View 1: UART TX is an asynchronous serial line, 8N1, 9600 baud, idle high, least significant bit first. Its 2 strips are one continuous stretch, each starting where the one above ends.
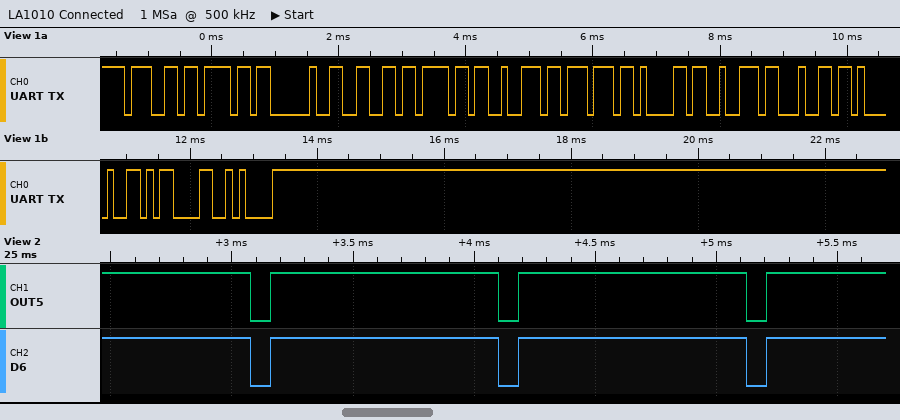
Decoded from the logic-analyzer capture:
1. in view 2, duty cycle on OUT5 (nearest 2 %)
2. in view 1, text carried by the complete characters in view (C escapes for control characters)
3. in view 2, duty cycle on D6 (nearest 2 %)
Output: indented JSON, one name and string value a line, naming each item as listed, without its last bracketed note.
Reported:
{
  "in view 2, duty cycle on OUT5": "92 %",
  "in view 1, text carried by the complete characters in view": "\"go forward!\\r\\n\"",
  "in view 2, duty cycle on D6": "92 %"
}
